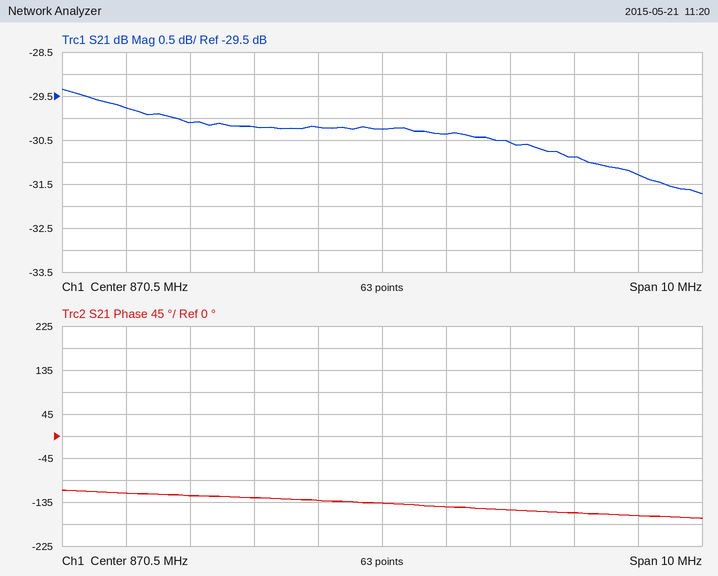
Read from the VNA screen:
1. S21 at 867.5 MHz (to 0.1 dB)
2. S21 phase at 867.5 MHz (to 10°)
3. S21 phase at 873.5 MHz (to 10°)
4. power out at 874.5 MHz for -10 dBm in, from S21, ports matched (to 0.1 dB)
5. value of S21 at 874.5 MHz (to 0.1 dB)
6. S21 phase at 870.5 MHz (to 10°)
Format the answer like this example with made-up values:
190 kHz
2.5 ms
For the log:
-30.1 dB
-120°
-160°
-41.3 dBm
-31.3 dB
-140°
